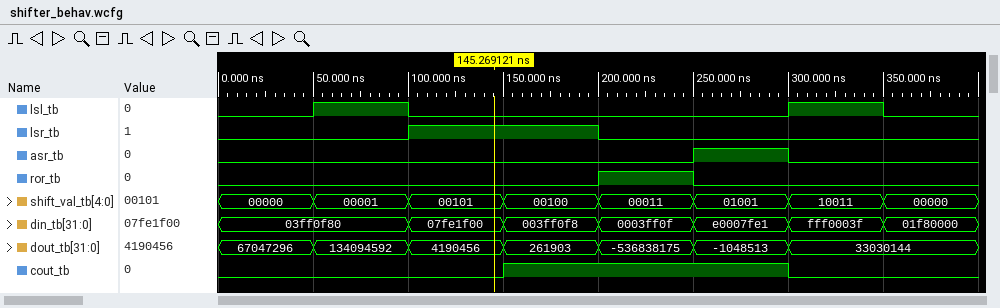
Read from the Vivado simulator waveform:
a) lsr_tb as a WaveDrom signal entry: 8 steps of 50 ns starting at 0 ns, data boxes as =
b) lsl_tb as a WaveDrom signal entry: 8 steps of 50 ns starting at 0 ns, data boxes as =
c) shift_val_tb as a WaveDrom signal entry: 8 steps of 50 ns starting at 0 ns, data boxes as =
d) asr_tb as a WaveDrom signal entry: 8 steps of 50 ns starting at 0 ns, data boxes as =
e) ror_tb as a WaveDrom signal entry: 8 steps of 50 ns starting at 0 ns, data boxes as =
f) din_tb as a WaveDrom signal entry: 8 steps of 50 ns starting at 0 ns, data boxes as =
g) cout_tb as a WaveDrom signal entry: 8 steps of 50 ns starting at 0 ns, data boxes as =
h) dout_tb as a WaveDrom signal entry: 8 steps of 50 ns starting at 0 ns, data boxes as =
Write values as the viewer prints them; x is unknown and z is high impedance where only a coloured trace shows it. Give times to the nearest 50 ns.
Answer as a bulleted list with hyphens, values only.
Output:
- {name: 'lsr_tb', wave: '0.1.0...'}
- {name: 'lsl_tb', wave: '010...10'}
- {name: 'shift_val_tb', wave: '========', data: '00000 00001 00101 00100 00011 01001 10011 00000'}
- {name: 'asr_tb', wave: '0....10.'}
- {name: 'ror_tb', wave: '0...10..'}
- {name: 'din_tb', wave: '=.======', data: '03ff0f80 07fe1f00 003ff0f8 0003ff0f e0007fe1 fff0003f 01f80000'}
- {name: 'cout_tb', wave: '0..1..0.'}
- {name: 'dout_tb', wave: '=======.', data: '67047296 134094592 4190456 261903 -536838175 -1048513 33030144'}
